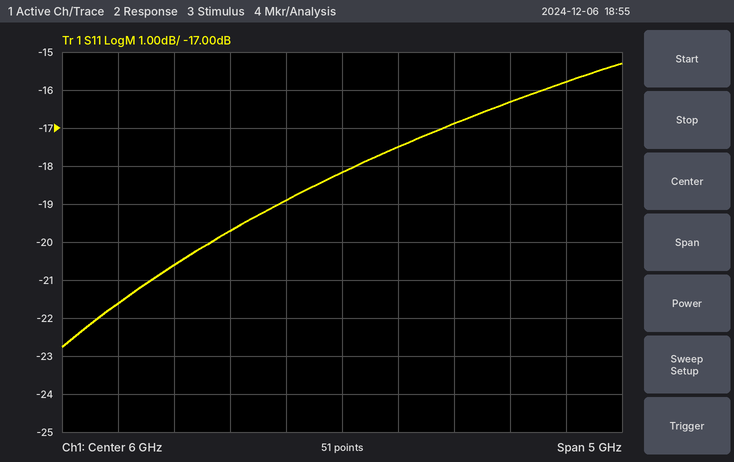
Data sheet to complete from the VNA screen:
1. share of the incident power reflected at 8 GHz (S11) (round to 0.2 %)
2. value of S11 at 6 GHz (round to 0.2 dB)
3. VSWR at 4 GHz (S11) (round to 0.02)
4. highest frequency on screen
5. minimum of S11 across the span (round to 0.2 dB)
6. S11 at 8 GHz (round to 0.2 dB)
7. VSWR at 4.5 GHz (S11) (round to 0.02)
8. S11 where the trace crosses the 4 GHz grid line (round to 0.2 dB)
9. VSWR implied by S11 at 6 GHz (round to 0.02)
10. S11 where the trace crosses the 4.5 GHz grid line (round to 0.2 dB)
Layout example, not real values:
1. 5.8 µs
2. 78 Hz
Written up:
1. 2.6 %
2. -18.2 dB
3. 1.18
4. 8.5 GHz
5. -22.8 dB
6. -15.8 dB
7. 1.20
8. -21.6 dB
9. 1.28
10. -20.6 dB
